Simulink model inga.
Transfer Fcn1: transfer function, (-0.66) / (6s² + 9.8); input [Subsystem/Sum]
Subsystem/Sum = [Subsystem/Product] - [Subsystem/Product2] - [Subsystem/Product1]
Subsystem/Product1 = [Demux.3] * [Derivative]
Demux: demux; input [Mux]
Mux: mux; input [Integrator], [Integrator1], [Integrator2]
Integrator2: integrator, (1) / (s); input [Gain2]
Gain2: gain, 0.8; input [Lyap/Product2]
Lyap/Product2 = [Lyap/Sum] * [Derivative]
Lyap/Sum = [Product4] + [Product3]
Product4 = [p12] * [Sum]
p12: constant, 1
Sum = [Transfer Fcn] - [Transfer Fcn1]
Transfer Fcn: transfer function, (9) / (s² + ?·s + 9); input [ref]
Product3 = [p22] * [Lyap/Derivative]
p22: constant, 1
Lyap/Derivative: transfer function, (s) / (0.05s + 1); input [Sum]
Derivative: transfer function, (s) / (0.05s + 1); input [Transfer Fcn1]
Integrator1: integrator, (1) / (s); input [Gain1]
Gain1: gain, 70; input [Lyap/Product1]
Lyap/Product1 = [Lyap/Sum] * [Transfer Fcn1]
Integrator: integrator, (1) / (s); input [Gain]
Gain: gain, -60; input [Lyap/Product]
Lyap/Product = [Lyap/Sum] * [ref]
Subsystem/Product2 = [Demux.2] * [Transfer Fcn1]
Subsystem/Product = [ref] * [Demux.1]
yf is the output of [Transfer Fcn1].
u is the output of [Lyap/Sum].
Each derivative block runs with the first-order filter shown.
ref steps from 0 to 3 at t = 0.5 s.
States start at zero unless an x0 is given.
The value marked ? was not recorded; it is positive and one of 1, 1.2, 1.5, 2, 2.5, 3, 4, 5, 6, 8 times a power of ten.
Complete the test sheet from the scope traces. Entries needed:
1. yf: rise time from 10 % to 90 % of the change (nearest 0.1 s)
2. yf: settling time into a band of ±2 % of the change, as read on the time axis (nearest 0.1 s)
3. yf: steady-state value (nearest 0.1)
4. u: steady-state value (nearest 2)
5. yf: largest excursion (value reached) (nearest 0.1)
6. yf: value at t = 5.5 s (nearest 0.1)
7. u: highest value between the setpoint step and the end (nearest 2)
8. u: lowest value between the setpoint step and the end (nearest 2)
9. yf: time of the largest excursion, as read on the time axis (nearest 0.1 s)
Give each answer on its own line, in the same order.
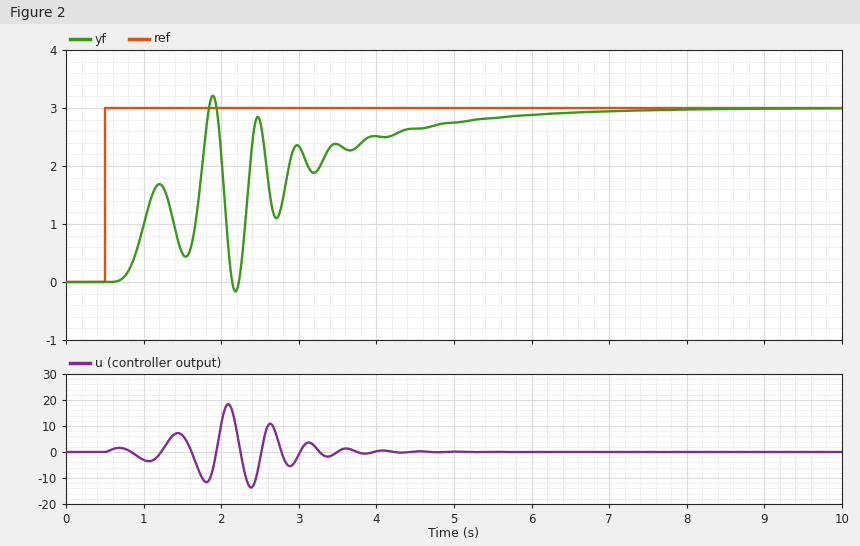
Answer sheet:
1.0 s
6.9 s
3.0
0
3.2
2.8
18
-14
1.9 s
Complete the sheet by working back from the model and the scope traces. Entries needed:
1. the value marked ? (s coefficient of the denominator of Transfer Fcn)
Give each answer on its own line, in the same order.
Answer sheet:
12
